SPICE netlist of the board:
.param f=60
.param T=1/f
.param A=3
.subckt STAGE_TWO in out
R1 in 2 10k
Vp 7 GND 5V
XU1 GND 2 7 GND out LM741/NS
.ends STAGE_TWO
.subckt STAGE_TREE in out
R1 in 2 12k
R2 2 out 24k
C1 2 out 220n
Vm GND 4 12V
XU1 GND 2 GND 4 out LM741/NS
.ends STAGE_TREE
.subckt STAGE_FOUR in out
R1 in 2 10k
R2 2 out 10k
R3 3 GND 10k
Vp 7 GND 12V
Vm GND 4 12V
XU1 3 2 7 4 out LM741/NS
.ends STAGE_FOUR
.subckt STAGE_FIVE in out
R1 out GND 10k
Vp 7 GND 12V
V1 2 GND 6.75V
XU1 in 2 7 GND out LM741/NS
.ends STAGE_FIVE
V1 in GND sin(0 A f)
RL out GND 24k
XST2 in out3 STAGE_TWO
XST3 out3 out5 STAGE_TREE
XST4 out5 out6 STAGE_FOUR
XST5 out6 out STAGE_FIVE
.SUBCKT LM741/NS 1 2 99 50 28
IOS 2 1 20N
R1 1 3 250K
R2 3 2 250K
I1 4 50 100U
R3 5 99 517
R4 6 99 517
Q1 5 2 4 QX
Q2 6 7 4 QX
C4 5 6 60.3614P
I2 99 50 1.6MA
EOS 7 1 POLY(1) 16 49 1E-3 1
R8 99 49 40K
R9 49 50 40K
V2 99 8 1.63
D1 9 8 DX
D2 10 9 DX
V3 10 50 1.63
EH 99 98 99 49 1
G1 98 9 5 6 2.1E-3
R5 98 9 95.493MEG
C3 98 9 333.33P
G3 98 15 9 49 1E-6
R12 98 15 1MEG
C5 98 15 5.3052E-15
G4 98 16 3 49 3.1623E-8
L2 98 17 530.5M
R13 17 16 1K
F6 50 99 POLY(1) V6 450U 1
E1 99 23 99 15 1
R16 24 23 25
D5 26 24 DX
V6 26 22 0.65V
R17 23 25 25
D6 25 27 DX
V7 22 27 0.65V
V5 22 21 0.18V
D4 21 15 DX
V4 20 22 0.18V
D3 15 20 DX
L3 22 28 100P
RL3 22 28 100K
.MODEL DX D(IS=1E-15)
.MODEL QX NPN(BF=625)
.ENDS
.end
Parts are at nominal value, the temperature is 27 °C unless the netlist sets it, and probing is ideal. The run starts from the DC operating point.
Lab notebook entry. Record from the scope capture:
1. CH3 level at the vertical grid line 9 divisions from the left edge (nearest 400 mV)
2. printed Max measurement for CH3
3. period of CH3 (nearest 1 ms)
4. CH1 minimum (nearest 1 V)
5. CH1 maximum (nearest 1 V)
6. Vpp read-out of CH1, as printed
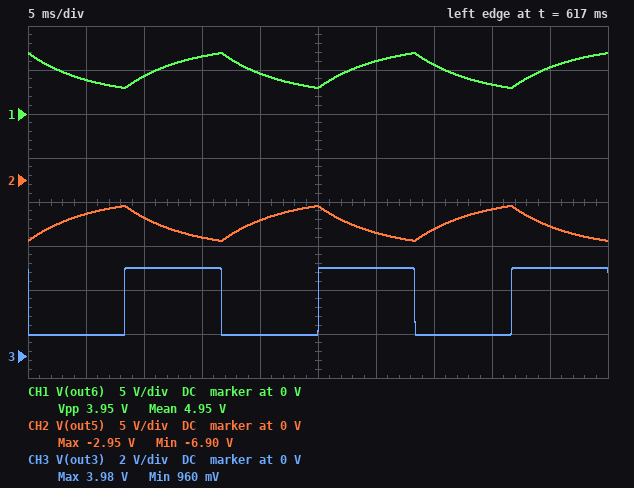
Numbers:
4.0 V
3.98 V
17 ms
3 V
7 V
3.95 V
